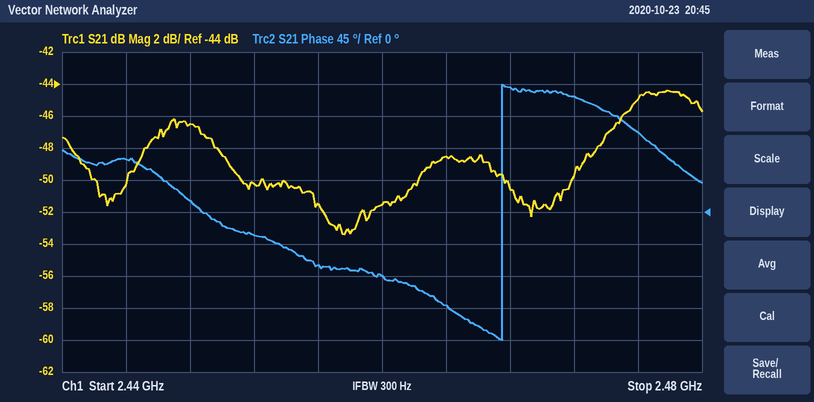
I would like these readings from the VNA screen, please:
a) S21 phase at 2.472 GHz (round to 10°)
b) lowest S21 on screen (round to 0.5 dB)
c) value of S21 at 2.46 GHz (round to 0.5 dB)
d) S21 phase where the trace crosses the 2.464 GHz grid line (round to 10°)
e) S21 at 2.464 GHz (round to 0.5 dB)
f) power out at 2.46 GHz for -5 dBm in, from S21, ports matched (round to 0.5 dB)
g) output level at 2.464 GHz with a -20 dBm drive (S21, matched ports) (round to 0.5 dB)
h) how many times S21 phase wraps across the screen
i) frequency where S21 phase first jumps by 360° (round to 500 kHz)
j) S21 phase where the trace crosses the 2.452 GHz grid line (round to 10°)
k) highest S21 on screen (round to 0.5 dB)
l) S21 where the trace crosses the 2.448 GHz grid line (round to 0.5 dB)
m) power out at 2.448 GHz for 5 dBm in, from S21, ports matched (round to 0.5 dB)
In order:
160°
-53.5 dB
-51.5 dB
-130°
-48.5 dB
-56.5 dBm
-68.5 dBm
1
2.4675 GHz
-30°
-44.5 dB
-46.5 dB
-41.5 dBm
